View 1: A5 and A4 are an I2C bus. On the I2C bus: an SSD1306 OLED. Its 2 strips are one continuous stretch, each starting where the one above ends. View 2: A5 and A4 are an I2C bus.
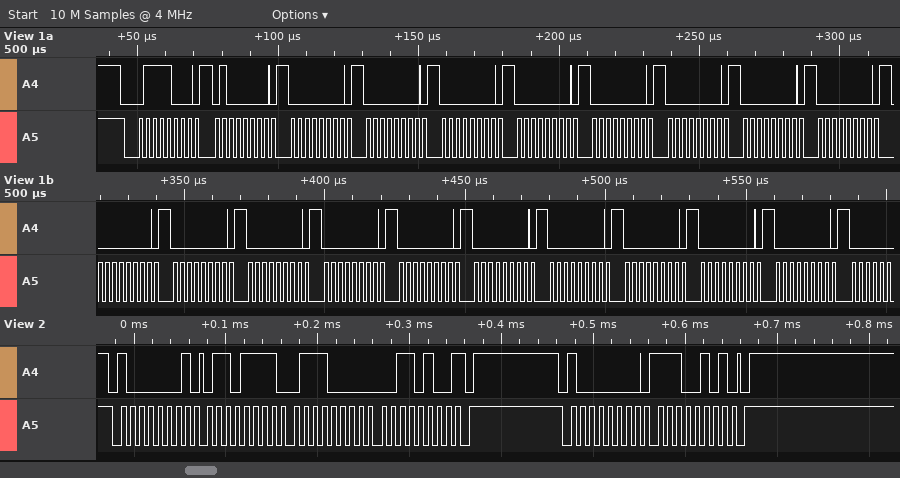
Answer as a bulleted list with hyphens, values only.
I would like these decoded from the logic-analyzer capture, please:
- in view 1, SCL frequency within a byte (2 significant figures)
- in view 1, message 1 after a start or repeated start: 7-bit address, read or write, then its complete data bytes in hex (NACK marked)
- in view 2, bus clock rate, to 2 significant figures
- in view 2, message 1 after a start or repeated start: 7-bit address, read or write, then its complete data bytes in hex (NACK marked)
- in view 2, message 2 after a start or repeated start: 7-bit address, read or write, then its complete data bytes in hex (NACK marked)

- 400 kHz
- 0x3C write: 40 00 00 00 00 00 00 00 00 00 00 00 00 00 00 00 00 00 00
- 100 kHz
- 0x40 read: 6F 70 34 NACK
- 0x40 write: E5
